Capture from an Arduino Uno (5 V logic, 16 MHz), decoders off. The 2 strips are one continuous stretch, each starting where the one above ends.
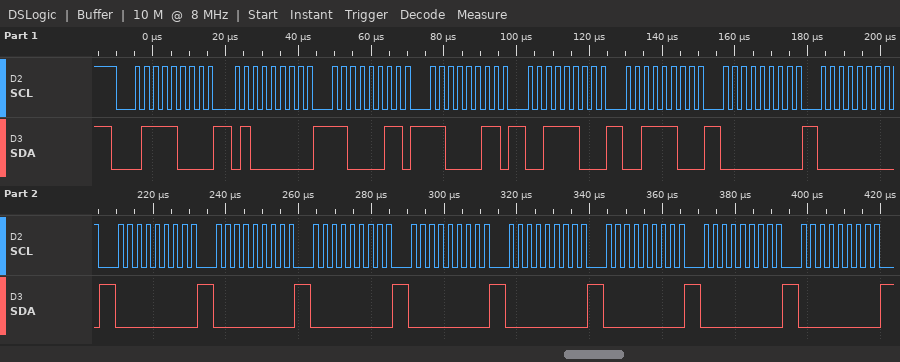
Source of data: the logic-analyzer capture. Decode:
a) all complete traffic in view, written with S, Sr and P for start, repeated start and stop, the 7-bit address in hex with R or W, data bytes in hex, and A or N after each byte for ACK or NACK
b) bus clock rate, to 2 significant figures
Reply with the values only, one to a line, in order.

S 3CW A 40 A C3 A C3 A 3C A 3C A 00 A 00 A 00 A 00 A 00 A 00 A 00 A 00 A 00 A 00 A
400 kHz
